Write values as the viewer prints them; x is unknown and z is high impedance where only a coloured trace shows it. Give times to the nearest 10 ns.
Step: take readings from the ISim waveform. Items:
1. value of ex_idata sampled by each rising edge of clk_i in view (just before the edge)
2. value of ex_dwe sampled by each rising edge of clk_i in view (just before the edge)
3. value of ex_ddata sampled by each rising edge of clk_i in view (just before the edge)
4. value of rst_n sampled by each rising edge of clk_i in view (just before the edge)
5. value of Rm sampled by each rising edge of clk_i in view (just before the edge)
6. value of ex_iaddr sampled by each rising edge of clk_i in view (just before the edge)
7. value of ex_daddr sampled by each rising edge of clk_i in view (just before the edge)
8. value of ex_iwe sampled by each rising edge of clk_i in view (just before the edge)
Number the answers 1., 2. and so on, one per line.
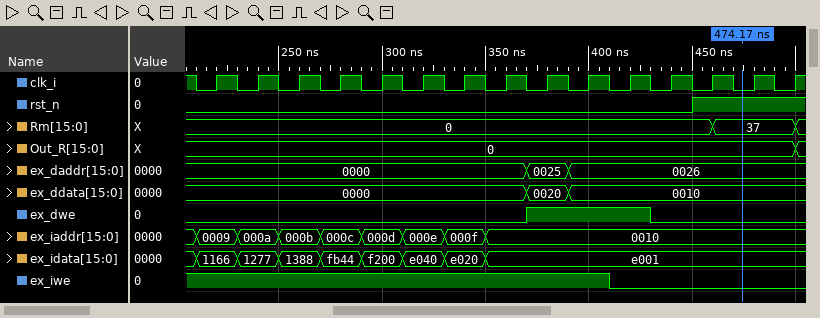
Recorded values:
1. 1166, 1277, 1388, fb44, f200, e040, e020, e001, e001, e001, e001, e001, e001, e001, e001
2. 0 0 0 0 0 0 0 0 1 1 1 0 0 0 0
3. 0000, 0000, 0000, 0000, 0000, 0000, 0000, 0000, 0020, 0010, 0010, 0010, 0010, 0010, 0010
4. 0 0 0 0 0 0 0 0 0 0 0 0 1 1 1
5. 0, 0, 0, 0, 0, 0, 0, 0, 0, 0, 0, 0, 0, 37, 37
6. 0009, 000a, 000b, 000c, 000d, 000e, 000f, 0010, 0010, 0010, 0010, 0010, 0010, 0010, 0010
7. 0000, 0000, 0000, 0000, 0000, 0000, 0000, 0000, 0025, 0026, 0026, 0026, 0026, 0026, 0026
8. 1 1 1 1 1 1 1 1 1 1 0 0 0 0 0
